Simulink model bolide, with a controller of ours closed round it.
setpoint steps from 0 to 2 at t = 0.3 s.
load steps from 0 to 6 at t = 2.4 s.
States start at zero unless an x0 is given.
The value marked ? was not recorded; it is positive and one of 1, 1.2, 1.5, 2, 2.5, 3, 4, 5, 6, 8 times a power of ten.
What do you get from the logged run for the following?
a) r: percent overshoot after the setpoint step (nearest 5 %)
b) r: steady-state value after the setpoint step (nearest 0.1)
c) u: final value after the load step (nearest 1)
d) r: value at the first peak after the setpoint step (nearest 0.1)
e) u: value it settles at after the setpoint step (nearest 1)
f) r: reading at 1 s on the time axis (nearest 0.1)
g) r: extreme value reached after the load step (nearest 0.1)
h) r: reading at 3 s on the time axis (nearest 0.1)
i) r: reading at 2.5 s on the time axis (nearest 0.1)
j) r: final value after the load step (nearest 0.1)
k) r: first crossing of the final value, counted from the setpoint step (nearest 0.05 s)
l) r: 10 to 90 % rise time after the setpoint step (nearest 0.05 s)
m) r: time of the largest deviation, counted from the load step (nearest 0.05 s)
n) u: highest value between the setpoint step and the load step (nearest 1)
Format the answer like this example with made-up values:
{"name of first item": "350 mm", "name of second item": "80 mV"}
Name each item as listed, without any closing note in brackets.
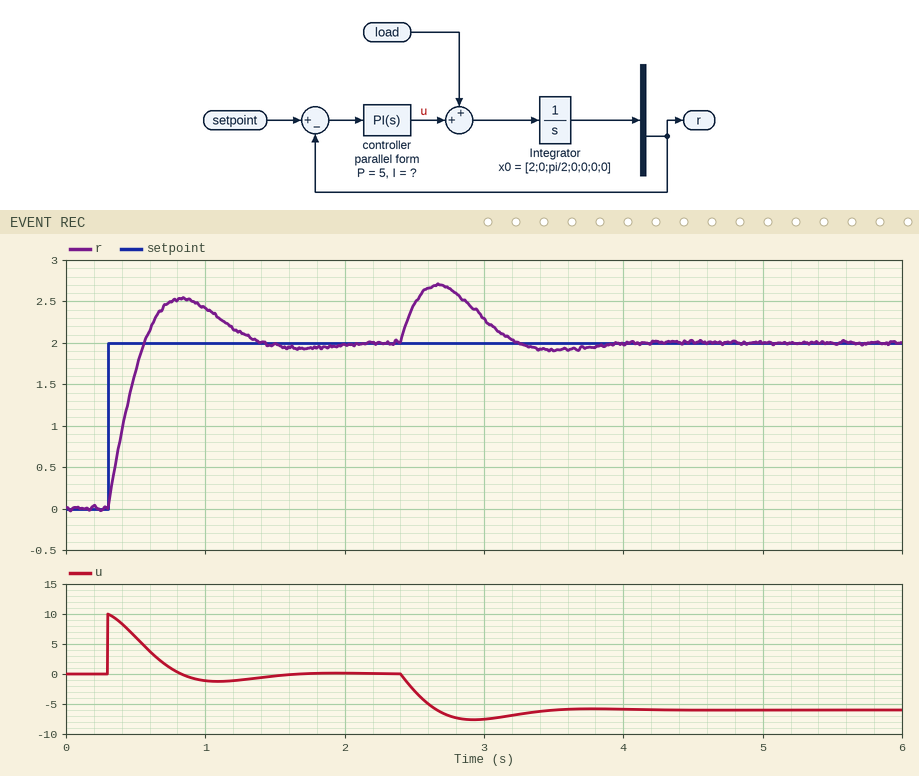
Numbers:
{"r: percent overshoot after the setpoint step": "25 %", "r: steady-state value after the setpoint step": "2.0", "u: final value after the load step": "-6", "r: value at the first peak after the setpoint step": "2.5", "u: value it settles at after the setpoint step": "0", "r: reading at 1 s on the time axis": "2.4", "r: extreme value reached after the load step": "2.7", "r: reading at 3 s on the time axis": "2.3", "r: reading at 2.5 s on the time axis": "2.5", "r: final value after the load step": "2.0", "r: first crossing of the final value, counted from the setpoint step": "0.25 s", "r: 10 to 90 % rise time after the setpoint step": "0.20 s", "r: time of the largest deviation, counted from the load step": "0.25 s", "u: highest value between the setpoint step and the load step": "10"}
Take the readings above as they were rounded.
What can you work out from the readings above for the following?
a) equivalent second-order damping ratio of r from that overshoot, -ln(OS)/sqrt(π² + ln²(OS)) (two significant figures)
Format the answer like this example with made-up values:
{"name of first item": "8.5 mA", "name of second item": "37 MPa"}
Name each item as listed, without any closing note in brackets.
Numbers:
{"equivalent second-order damping ratio of r from that overshoot, -ln(OS)/sqrt(π² + ln²(OS))": "0.40"}
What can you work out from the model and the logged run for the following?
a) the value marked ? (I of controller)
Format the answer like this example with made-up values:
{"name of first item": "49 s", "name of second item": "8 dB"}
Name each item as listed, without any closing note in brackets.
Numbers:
{"the value marked ?": "20"}
